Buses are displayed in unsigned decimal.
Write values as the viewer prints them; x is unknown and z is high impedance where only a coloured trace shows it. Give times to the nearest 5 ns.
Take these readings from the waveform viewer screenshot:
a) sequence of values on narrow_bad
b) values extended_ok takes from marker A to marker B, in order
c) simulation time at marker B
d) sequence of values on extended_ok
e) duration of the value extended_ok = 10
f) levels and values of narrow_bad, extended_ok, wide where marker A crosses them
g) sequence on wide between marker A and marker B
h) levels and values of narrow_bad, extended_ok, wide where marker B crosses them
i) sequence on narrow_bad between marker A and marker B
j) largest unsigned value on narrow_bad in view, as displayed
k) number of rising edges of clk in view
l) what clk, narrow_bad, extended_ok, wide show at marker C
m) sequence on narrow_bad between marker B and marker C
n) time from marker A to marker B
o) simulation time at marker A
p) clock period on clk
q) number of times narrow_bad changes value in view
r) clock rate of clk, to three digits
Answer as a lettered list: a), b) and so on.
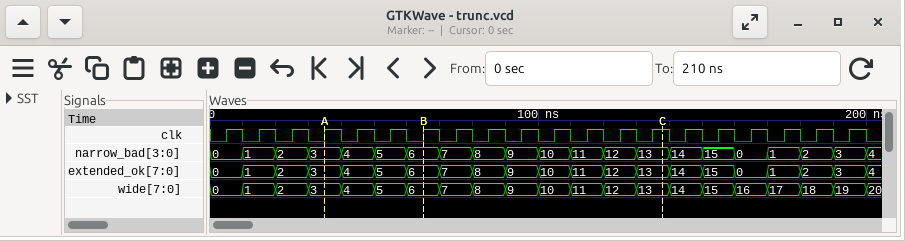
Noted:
a) 0, 1, 2, 3, 4, 5, 6, 7, 8, 9, 10, 11, 12, 13, 14, 15, 0, 1, 2, 3, 4
b) 3, 4, 5, 6
c) 65 ns
d) 0, 1, 2, 3, 4, 5, 6, 7, 8, 9, 10, 11, 12, 13, 14, 15, 0, 1, 2, 3, 4
e) 10 ns
f) narrow_bad=3, extended_ok=3, wide=3
g) 3, 4, 5, 6
h) narrow_bad=6, extended_ok=6, wide=6
i) 3, 4, 5, 6
j) 15
k) 20
l) clk=1, narrow_bad=13, extended_ok=13, wide=13
m) 6, 7, 8, 9, 10, 11, 12, 13
n) 30 ns
o) 35 ns
p) 10 ns
q) 20
r) 100 MHz
